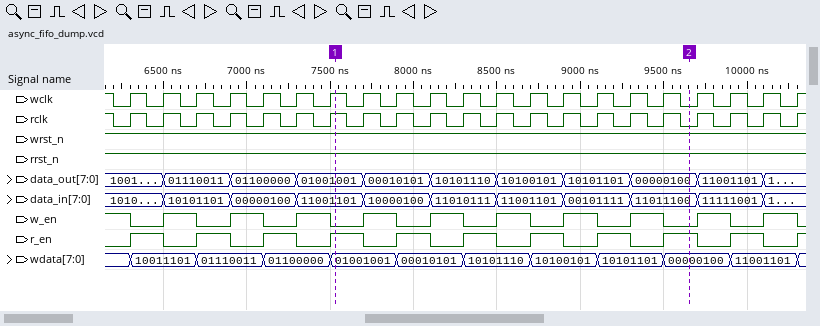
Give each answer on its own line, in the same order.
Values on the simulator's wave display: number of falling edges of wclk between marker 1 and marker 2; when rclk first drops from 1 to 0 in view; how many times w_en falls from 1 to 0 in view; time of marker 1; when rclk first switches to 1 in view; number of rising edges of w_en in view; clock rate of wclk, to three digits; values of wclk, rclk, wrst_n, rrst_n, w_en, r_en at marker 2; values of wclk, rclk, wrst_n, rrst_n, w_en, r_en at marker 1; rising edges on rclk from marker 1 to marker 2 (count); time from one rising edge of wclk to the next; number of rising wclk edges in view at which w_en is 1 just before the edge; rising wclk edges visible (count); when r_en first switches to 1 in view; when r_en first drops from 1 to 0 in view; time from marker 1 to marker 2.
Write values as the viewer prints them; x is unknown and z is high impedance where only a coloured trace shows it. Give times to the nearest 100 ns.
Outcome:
11
6200 ns
11
7500 ns
6300 ns
10
5.00 MHz
wclk=0, rclk=0, wrst_n=1, rrst_n=1, w_en=0, r_en=1
wclk=1, rclk=1, wrst_n=1, rrst_n=1, w_en=0, r_en=1
10
200 ns
11
21
6300 ns
6500 ns
2100 ns
